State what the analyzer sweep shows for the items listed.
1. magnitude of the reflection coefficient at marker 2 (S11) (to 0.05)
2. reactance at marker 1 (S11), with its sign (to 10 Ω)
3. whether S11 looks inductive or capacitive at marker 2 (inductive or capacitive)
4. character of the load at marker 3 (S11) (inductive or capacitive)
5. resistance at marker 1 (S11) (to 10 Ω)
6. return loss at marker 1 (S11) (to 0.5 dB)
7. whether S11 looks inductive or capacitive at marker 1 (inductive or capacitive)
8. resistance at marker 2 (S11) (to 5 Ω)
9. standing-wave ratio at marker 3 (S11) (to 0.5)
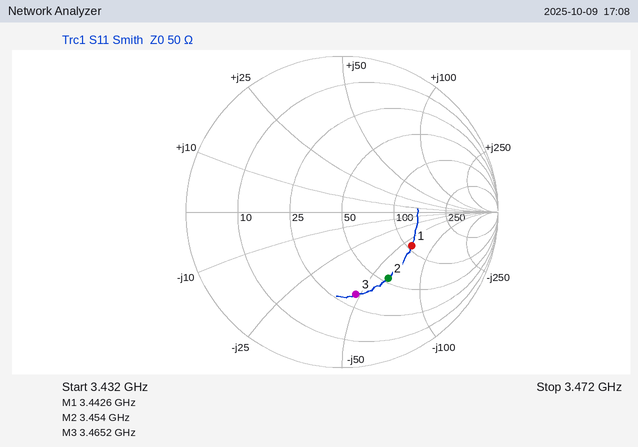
0.50
-60 Ω
capacitive
capacitive
110 Ω
6.0 dB
capacitive
55 Ω
3.5
